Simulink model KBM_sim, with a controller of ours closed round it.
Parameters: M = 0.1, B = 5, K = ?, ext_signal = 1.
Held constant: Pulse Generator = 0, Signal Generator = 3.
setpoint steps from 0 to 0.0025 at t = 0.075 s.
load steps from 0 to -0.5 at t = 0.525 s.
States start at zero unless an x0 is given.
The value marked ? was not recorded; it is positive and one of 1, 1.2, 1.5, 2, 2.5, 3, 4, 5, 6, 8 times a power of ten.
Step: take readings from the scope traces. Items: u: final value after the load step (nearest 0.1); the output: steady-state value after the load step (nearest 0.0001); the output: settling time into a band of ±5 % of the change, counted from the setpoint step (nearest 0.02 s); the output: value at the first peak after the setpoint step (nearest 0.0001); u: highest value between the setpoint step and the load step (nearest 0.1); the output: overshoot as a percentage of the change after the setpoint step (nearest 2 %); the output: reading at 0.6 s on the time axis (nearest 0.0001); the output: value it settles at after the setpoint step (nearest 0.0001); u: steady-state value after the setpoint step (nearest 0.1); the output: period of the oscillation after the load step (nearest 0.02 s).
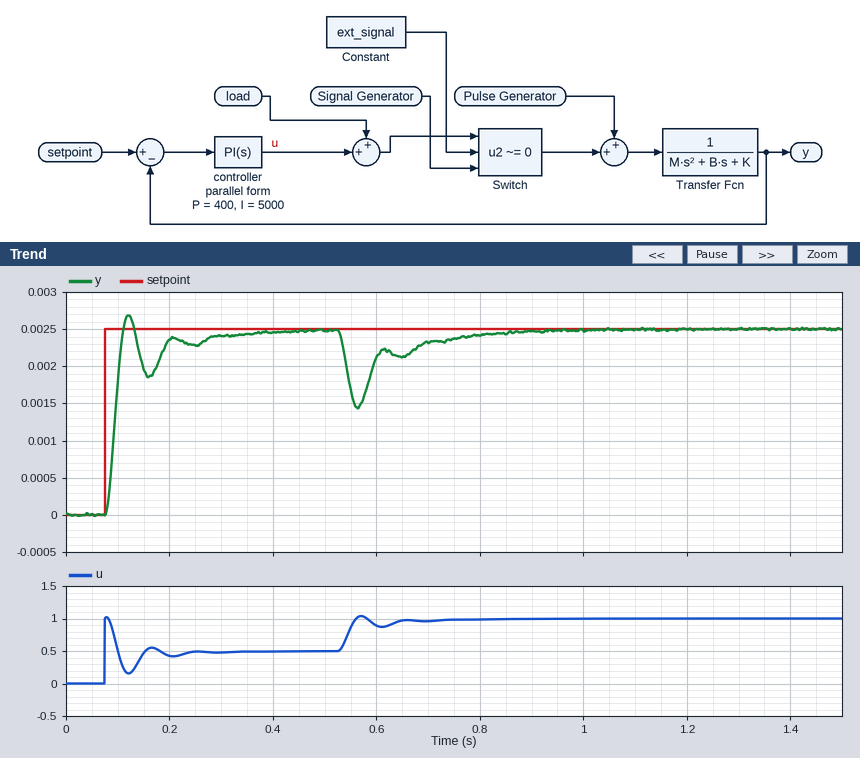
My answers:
1.0
0.0025
0.20 s
0.0027
1.0
8 %
0.0021
0.0025
0.5
0.08 s
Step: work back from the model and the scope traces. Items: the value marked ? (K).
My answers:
200
